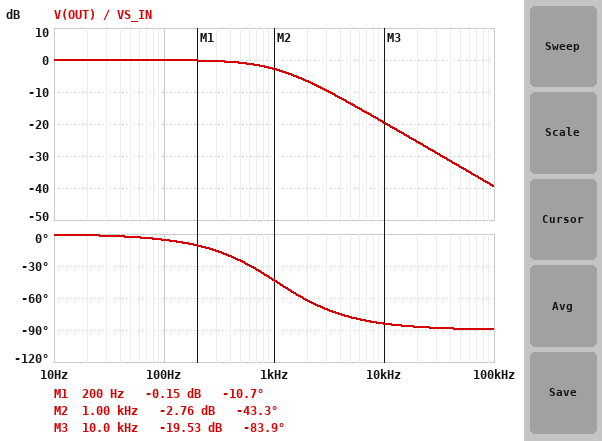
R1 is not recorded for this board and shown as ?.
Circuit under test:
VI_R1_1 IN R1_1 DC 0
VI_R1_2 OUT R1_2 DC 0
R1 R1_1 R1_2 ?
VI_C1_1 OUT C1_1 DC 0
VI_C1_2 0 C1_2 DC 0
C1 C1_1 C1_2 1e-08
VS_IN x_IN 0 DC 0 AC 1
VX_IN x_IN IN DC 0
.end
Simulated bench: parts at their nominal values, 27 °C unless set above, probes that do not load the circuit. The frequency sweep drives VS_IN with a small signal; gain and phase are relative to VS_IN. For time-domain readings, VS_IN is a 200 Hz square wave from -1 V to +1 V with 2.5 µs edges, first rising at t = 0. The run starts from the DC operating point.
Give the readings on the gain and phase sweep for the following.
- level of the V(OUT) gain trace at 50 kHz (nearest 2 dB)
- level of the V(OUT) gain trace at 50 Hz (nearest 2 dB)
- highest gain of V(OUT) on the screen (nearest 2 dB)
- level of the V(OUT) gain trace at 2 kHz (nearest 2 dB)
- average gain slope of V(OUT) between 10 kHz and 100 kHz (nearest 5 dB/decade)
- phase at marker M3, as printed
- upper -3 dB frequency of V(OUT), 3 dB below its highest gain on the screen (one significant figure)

-34 dB
0 dB
0 dB
-6 dB
-20 dB/decade
-83.9 deg
1 kHz
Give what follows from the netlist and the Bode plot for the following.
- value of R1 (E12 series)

15 kΩ
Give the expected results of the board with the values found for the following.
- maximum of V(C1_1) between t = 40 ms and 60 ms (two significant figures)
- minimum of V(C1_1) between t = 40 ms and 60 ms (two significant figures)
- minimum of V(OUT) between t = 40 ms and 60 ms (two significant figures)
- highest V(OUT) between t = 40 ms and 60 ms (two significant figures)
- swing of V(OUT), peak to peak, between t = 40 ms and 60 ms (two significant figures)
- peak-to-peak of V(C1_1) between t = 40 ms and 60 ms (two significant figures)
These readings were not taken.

1.0 V
-1.0 V
-1.0 V
1.0 V
2.0 V
2.0 V
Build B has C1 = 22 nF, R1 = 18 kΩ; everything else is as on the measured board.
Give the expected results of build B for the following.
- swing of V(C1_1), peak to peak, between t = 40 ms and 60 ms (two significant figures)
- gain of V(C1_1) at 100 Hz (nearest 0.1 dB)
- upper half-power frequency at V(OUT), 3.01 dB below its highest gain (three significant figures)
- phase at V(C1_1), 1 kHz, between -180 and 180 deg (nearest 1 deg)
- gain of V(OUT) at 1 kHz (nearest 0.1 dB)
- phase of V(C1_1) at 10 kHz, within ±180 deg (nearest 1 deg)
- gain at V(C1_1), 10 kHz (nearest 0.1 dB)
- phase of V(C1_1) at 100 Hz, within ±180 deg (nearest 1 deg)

2.0 V
-0.3 dB
402 Hz
-68 deg
-8.6 dB
-88 deg
-27.9 dB
-14 deg
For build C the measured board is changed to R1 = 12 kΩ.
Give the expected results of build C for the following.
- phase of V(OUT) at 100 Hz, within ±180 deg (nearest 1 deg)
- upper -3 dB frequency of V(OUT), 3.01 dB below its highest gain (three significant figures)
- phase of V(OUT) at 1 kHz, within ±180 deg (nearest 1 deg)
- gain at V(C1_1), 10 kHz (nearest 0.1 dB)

-4 deg
1.33 kHz
-37 deg
-17.6 dB
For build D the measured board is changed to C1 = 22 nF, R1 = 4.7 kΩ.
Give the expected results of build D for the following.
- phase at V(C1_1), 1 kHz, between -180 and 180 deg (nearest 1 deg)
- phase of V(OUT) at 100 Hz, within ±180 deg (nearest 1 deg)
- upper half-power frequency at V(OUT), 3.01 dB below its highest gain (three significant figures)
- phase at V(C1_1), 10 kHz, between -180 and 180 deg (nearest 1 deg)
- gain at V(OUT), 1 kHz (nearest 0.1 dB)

-33 deg
-4 deg
1.54 kHz
-81 deg
-1.5 dB
